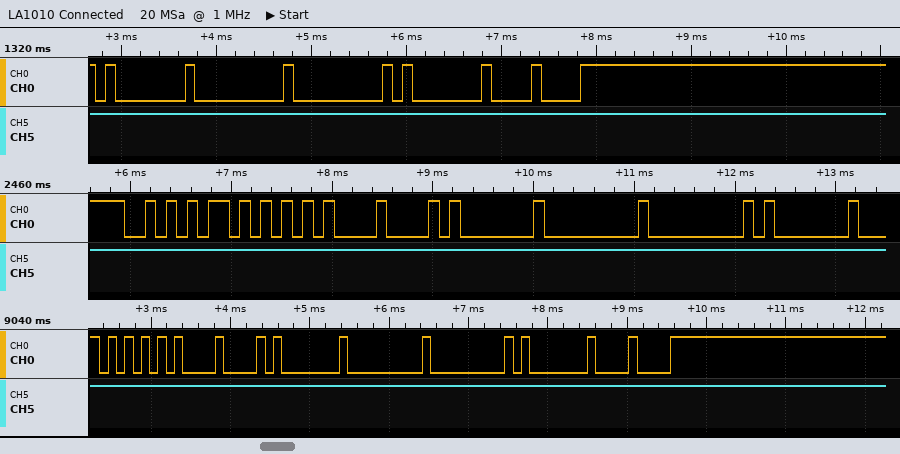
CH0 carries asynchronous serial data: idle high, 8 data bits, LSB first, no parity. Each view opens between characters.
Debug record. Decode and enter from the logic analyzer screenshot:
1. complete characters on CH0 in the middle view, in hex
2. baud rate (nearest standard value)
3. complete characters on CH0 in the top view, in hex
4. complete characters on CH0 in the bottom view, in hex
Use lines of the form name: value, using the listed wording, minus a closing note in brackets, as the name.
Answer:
complete characters on CH0 in the middle view, in hex: AA, 55, 08, 01, 00, 00, 01
baud rate: 9600 baud
complete characters on CH0 in the top view, in hex: 01, 00, 00, 01, 08
complete characters on CH0 in the bottom view, in hex: 55, 08, 01, 00, 00, 01, 08
